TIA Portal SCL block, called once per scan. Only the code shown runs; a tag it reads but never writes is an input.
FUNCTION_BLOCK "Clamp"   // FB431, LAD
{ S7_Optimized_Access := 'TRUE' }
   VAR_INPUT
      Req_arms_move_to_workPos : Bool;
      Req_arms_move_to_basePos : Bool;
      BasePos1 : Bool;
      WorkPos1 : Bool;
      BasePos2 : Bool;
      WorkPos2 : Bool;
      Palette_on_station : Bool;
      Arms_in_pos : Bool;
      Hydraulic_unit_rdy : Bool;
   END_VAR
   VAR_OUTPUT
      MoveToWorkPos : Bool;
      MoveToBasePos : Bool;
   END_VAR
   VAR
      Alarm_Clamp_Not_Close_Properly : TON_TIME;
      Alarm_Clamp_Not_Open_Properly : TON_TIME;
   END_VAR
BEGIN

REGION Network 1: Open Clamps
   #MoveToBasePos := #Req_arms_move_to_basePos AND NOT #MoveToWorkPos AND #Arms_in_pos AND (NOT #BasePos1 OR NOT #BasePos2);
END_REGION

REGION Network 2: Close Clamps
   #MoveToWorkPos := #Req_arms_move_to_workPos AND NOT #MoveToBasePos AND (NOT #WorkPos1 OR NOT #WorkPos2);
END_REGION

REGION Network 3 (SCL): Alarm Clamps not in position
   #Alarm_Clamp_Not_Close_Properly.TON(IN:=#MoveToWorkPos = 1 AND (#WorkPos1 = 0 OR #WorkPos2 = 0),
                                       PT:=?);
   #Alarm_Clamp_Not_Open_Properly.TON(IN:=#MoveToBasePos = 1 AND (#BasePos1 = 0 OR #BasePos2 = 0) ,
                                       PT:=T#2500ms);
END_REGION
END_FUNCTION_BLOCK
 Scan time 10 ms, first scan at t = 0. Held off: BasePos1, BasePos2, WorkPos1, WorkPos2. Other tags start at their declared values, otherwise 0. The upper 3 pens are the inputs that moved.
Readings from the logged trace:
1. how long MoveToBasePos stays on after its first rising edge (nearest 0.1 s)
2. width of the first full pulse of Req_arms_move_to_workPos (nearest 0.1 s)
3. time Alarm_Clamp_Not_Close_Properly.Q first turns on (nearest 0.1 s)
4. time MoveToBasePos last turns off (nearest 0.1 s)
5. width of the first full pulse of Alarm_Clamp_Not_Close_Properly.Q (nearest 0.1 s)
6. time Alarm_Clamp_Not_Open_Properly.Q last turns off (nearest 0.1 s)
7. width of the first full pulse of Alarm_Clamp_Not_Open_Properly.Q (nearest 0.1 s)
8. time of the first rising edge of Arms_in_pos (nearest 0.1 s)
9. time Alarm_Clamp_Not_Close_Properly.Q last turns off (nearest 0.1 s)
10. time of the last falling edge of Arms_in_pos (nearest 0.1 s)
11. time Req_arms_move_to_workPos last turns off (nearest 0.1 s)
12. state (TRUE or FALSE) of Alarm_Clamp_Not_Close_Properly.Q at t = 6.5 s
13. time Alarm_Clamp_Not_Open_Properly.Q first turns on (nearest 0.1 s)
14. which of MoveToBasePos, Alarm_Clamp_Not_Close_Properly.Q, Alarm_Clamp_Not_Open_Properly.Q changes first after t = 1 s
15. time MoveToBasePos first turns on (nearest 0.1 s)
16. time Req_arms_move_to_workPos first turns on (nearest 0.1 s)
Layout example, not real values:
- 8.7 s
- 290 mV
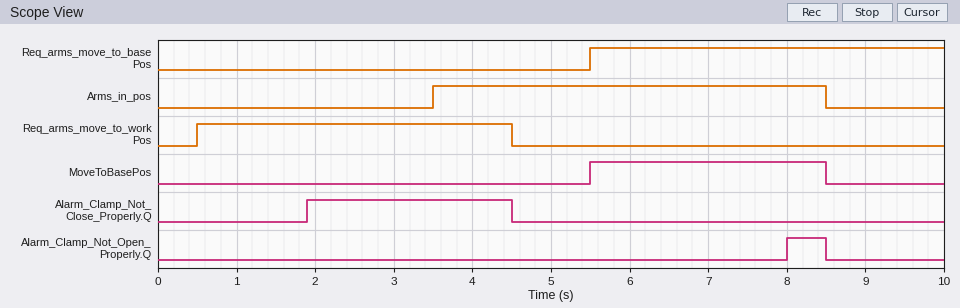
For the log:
- 3.0 s
- 4.0 s
- 1.9 s
- 8.5 s
- 2.6 s
- 8.5 s
- 0.5 s
- 3.5 s
- 4.5 s
- 8.5 s
- 4.5 s
- FALSE
- 8.0 s
- Alarm_Clamp_Not_Close_Properly.Q
- 5.5 s
- 0.5 s
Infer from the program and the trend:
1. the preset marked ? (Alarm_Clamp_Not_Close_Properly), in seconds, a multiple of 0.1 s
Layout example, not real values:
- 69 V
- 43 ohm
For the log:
- 1.4 s
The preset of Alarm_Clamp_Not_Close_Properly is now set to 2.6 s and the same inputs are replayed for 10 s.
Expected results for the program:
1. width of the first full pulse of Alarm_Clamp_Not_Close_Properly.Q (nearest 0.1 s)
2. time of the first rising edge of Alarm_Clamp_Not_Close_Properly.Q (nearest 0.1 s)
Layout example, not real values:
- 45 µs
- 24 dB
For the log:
- 1.4 s
- 3.1 s
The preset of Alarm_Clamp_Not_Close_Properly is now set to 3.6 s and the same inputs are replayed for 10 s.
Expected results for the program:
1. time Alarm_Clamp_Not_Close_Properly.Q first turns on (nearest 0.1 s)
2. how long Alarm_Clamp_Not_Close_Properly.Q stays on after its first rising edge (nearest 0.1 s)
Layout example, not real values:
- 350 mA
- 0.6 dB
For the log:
- 4.1 s
- 0.4 s
